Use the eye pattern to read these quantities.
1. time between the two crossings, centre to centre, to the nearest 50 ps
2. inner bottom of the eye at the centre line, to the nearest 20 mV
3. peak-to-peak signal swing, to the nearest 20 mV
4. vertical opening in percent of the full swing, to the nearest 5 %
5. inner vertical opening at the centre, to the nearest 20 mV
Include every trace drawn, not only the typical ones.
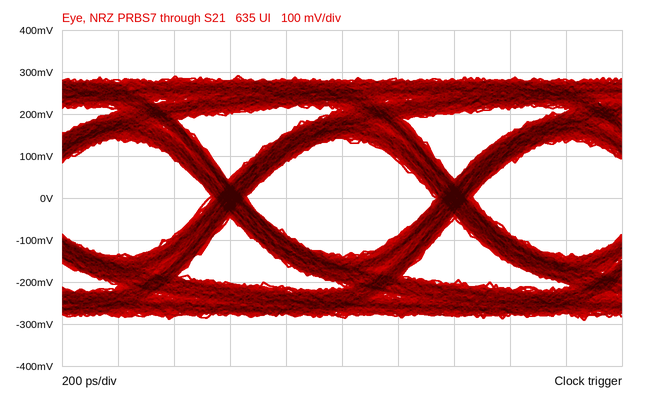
800 ps
-140 mV
580 mV
50 %
280 mV
